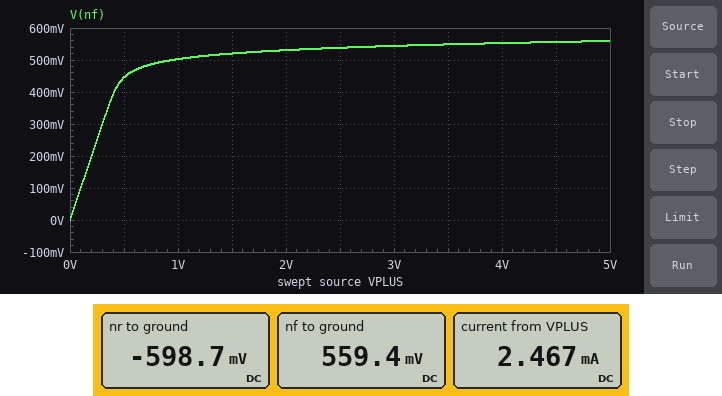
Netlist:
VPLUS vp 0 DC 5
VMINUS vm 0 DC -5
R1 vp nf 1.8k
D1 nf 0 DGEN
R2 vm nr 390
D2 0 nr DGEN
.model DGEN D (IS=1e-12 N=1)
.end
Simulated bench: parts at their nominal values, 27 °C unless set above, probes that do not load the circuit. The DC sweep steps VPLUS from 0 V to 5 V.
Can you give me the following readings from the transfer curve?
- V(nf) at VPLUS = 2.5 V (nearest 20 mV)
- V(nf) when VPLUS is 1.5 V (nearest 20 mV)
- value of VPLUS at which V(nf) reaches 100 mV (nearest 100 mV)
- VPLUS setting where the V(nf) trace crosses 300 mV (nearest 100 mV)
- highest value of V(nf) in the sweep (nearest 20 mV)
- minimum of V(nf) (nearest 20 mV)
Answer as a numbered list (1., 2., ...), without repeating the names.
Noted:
1. 540 mV
2. 520 mV
3. 100 mV
4. 300 mV
5. 560 mV
6. 0 V
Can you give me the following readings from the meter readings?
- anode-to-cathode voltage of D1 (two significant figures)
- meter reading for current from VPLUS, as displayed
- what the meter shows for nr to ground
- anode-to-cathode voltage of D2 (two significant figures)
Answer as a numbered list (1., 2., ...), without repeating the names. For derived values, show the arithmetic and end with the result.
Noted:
1. 559.4 mV = 560 mV
2. 2.467 mA
3. -598.7 mV
4. 0 V - (-598.7 mV) = 600 mV
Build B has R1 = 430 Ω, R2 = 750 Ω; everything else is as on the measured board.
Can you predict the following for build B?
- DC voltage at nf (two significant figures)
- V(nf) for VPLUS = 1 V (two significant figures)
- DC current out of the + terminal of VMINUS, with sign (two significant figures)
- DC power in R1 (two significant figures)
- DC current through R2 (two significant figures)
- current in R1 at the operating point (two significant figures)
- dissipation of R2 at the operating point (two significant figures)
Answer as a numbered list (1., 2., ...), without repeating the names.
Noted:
1. 600 mV
2. 540 mV
3. -5.9 mA
4. 45 mW
5. 5.9 mA
6. 10 mA
7. 26 mW
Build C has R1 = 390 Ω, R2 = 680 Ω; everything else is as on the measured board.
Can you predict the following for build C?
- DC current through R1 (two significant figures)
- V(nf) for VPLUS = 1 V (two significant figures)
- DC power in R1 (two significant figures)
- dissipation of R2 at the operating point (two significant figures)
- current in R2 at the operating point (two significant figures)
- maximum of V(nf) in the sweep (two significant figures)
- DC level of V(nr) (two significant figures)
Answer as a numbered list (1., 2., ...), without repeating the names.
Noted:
1. 11 mA
2. 540 mV
3. 50 mW
4. 29 mW
5. 6.5 mA
6. 600 mV
7. -580 mV
